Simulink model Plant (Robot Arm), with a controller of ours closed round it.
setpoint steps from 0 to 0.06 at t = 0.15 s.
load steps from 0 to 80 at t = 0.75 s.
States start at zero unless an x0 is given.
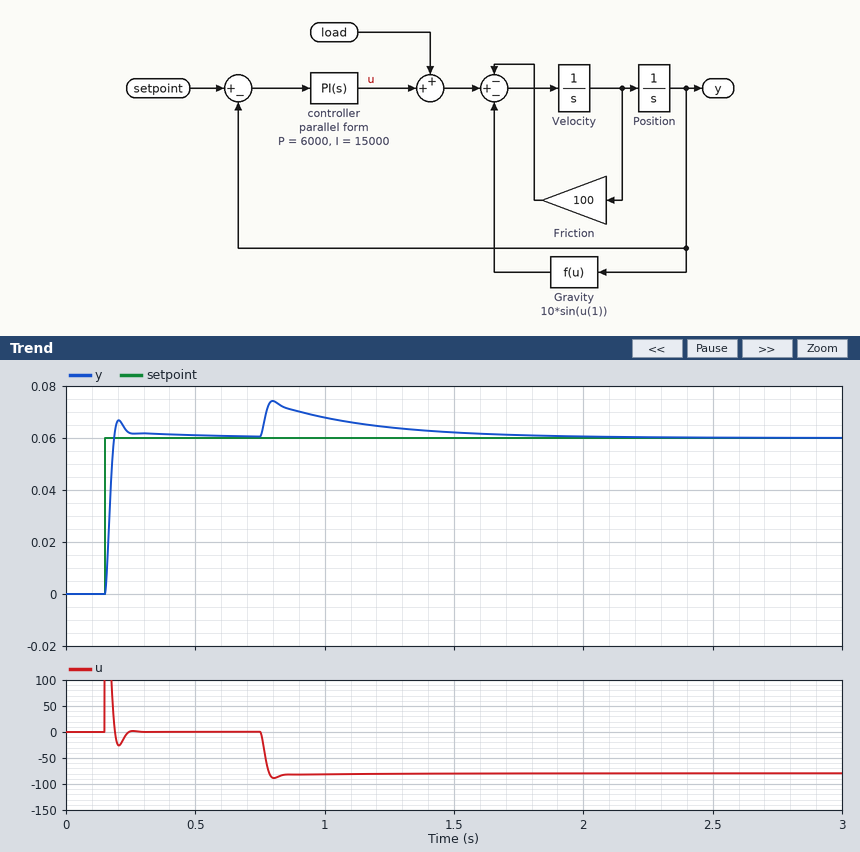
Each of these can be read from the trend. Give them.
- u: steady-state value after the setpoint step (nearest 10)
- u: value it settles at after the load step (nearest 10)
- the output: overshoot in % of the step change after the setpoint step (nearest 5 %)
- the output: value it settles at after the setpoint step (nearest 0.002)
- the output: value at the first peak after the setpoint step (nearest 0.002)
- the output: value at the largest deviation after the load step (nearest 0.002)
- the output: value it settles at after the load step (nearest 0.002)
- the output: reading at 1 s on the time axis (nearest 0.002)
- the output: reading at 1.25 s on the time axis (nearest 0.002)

0
-80
10 %
0.060
0.066
0.074
0.060
0.068
0.064
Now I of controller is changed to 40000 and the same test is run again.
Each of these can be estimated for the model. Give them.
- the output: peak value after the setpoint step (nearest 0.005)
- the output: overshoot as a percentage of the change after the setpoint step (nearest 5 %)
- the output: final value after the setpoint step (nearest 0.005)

0.070
20 %
0.060
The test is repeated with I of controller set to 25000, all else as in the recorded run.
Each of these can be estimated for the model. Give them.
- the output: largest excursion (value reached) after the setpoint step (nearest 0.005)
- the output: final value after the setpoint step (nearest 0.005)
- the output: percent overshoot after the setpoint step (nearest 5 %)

0.070
0.060
15 %
